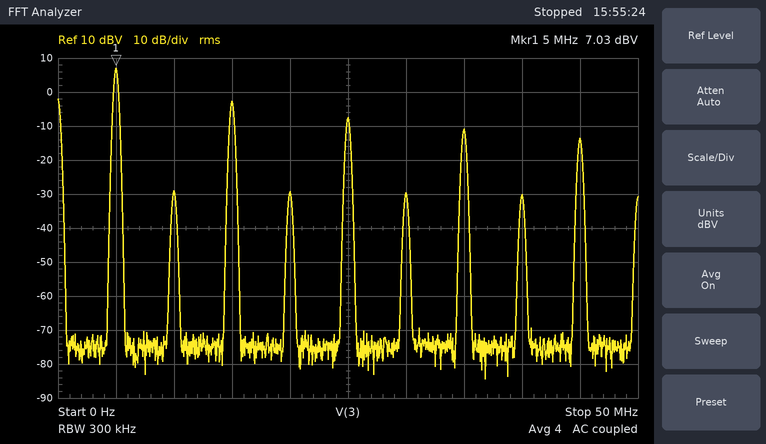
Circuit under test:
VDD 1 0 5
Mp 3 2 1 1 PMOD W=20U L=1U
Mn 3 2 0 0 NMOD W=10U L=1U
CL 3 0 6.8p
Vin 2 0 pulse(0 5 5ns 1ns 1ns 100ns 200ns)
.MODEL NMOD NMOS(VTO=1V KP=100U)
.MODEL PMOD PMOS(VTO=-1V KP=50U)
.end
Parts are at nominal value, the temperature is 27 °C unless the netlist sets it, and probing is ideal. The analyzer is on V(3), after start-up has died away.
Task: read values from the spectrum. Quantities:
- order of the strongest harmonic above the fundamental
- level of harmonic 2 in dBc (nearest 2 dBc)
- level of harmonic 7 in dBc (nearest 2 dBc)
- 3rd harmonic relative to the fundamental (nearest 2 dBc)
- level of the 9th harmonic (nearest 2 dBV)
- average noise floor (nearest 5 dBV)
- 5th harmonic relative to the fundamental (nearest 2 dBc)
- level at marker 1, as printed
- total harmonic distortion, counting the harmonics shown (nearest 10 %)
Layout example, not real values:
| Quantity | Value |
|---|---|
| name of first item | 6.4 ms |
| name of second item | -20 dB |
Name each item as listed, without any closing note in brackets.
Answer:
| Quantity | Value |
|---|---|
| order of the strongest harmonic above the fundamental | 3 |
| level of harmonic 2 in dBc | -36 dBc |
| level of harmonic 7 in dBc | -18 dBc |
| 3rd harmonic relative to the fundamental | -10 dBc |
| level of the 9th harmonic | -14 dBV |
| average noise floor | -75 dBV |
| 5th harmonic relative to the fundamental | -14 dBc |
| level at marker 1, as printed | 7.03 dBV |
| total harmonic distortion, counting the harmonics shown | 40 % |
